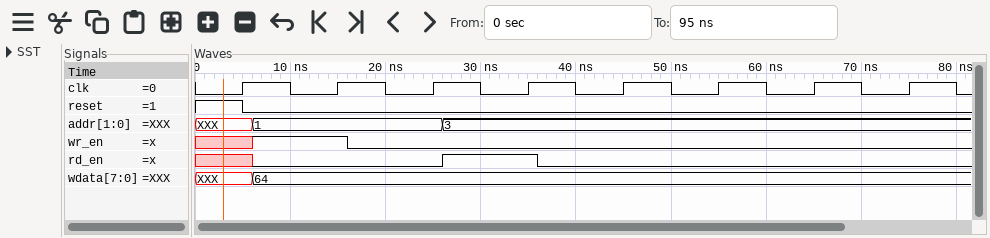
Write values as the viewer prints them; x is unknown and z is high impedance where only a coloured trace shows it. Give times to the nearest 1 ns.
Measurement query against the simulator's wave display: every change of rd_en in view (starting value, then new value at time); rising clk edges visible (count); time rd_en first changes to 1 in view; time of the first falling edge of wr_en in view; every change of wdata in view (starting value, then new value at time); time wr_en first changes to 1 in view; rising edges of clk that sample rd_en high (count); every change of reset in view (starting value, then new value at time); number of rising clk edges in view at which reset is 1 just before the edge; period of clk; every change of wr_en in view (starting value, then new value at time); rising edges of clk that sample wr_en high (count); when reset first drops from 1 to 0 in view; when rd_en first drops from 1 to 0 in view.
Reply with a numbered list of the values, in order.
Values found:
1. x, 0 at 6 ns, 1 at 26 ns, 0 at 36 ns
2. 8
3. 26 ns
4. 16 ns
5. XXX, 64 at 6 ns
6. 6 ns
7. 1
8. 1, 0 at 5 ns
9. 1
10. 10 ns
11. x, 1 at 6 ns, 0 at 16 ns
12. 1
13. 5 ns
14. 36 ns
